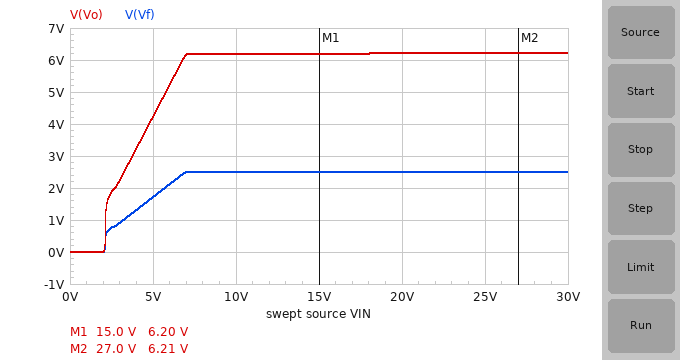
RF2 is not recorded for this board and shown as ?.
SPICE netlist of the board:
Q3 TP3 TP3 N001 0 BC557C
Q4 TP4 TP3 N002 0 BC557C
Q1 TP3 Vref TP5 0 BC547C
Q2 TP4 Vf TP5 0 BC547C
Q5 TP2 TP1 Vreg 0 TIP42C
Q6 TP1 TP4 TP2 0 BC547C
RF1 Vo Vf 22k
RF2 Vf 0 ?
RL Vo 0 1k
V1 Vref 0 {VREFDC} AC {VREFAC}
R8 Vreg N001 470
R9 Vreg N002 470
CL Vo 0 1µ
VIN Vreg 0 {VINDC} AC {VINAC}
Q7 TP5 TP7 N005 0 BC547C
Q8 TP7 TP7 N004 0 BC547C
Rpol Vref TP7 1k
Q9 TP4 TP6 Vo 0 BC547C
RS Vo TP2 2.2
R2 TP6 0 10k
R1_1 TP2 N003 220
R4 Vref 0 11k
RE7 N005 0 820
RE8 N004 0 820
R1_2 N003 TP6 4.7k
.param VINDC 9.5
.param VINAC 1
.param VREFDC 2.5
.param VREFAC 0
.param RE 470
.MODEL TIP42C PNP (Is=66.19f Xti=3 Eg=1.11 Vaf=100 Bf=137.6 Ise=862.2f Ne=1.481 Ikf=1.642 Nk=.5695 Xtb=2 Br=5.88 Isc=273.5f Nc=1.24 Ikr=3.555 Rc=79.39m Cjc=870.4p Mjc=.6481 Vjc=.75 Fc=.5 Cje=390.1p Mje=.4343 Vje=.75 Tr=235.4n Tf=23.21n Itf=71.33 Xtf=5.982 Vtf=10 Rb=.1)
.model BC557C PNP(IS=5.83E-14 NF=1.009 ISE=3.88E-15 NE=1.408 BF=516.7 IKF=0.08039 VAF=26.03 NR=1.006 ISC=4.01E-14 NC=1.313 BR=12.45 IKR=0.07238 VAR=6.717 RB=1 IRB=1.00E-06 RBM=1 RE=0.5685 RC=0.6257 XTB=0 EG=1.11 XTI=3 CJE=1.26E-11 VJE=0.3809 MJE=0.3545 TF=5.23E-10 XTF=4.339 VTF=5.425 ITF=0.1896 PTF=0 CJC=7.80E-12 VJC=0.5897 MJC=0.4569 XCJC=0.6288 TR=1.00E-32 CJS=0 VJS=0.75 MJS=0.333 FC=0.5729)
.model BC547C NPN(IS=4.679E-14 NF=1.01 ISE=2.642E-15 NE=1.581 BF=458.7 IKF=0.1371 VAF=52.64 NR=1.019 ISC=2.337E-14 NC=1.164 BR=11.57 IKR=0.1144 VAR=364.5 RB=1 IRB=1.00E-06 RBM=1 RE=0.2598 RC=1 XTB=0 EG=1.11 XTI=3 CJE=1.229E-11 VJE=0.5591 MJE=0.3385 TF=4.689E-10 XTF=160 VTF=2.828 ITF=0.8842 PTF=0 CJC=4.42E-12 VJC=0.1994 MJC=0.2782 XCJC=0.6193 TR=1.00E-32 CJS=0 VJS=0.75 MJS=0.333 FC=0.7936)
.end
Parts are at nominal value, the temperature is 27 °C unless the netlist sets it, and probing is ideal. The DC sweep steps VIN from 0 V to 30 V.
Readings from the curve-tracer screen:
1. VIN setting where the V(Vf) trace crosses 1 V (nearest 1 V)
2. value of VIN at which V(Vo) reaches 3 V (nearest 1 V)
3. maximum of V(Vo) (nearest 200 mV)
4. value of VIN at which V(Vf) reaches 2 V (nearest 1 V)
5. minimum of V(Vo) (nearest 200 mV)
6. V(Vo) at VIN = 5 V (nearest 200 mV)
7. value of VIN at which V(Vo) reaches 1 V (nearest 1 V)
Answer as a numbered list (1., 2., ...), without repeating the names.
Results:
1. 3 V
2. 4 V
3. 6.2 V
4. 6 V
5. 0 V
6. 4.2 V
7. 2 V
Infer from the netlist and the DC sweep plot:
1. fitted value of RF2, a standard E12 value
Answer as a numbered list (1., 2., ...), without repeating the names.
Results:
1. 15 kΩ
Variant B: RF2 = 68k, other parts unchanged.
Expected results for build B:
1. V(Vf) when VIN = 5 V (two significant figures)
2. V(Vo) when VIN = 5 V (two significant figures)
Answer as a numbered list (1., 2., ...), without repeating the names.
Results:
1. 2.5 V
2. 3.3 V
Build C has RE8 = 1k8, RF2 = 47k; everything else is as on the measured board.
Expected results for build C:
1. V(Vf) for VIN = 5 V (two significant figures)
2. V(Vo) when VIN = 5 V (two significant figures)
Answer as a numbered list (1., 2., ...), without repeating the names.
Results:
1. 2.5 V
2. 3.7 V
